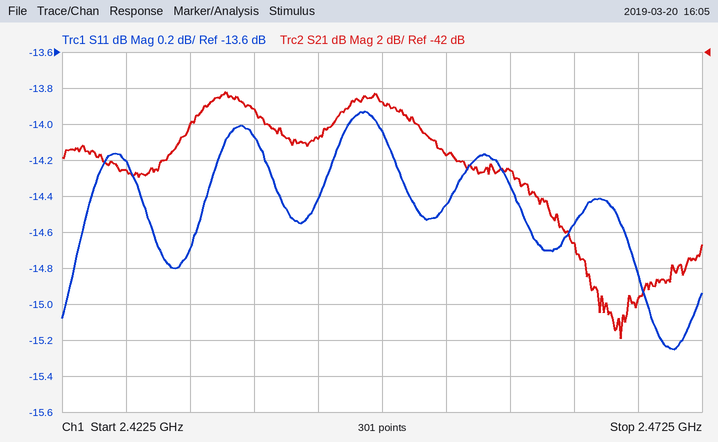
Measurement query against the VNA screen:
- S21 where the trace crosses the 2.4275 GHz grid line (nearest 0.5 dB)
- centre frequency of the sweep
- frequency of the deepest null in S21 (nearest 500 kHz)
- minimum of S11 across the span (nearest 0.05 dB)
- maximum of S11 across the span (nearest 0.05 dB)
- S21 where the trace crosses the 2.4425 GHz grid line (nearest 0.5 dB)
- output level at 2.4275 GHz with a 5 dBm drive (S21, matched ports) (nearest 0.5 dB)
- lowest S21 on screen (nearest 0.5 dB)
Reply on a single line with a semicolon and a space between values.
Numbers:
-48.5 dB; 2.4475 GHz; 2.4660 GHz; -15.25 dB; -13.95 dB; -47.0 dB; -43.5 dBm; -58.0 dB
